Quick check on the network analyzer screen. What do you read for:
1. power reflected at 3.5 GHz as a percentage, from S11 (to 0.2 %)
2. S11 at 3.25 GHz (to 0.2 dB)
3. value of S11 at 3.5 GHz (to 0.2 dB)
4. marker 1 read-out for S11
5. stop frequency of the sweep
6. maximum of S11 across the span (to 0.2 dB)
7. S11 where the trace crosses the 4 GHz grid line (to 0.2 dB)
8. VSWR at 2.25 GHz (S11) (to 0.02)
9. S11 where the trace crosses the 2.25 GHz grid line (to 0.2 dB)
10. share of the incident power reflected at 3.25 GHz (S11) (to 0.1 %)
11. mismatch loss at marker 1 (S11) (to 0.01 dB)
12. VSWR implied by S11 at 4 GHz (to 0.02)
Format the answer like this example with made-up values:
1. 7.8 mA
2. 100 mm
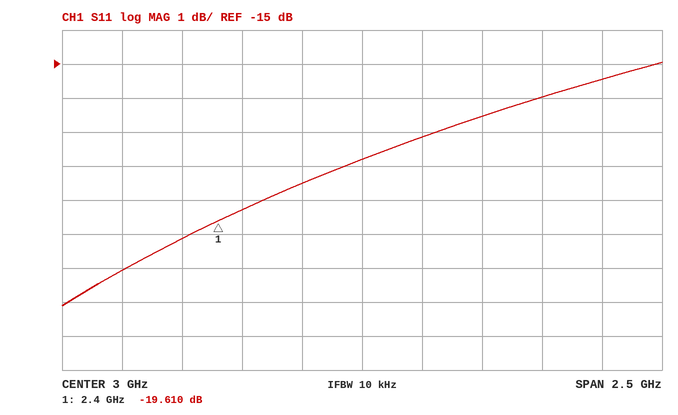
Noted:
1. 2.2 %
2. -17.2 dB
3. -16.6 dB
4. -19.610 dB
5. 4.25 GHz
6. -15.0 dB
7. -15.4 dB
8. 1.22
9. -20.2 dB
10. 1.9 %
11. 0.05 dB
12. 1.40
